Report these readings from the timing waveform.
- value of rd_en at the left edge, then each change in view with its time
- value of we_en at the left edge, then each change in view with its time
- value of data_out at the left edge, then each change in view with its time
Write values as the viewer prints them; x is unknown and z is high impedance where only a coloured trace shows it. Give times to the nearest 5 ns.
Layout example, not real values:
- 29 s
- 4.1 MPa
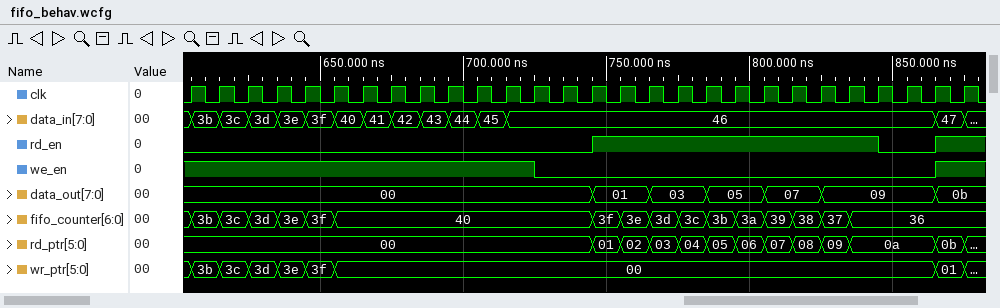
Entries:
- 0, 1 at 745 ns, 0 at 845 ns, 1 at 865 ns
- 1, 0 at 725 ns, 1 at 865 ns
- 00, 01 at 745 ns, 03 at 765 ns, 05 at 785 ns, 07 at 805 ns, 09 at 825 ns, 0b at 865 ns
